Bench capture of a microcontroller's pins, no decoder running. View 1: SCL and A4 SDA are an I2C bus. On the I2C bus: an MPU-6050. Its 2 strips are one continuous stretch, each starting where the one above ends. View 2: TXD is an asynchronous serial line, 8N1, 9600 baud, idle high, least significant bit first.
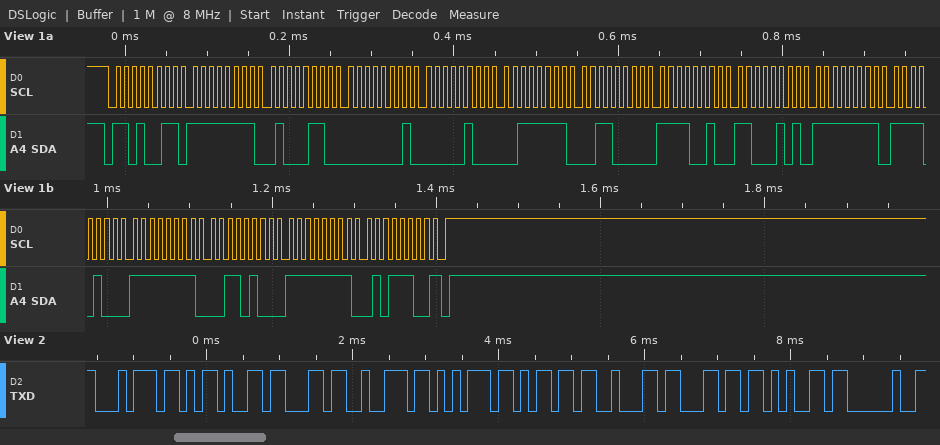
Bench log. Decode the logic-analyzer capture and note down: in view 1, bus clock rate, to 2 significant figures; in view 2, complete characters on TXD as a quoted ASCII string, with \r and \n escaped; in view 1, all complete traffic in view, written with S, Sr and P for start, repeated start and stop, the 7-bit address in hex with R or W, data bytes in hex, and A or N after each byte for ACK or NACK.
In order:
100 kHz
"t-crumble "
S 69R A FF A 46 A 01 A 04 A 3F A 30 A F2 A C5 A FF A F4 A FF A 34 A FF A 5C N P
